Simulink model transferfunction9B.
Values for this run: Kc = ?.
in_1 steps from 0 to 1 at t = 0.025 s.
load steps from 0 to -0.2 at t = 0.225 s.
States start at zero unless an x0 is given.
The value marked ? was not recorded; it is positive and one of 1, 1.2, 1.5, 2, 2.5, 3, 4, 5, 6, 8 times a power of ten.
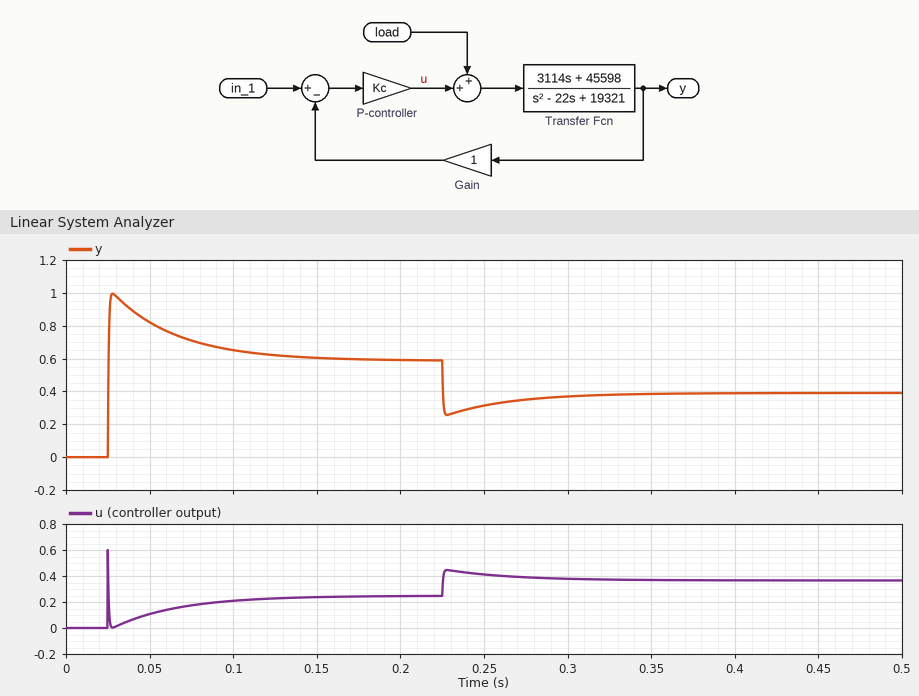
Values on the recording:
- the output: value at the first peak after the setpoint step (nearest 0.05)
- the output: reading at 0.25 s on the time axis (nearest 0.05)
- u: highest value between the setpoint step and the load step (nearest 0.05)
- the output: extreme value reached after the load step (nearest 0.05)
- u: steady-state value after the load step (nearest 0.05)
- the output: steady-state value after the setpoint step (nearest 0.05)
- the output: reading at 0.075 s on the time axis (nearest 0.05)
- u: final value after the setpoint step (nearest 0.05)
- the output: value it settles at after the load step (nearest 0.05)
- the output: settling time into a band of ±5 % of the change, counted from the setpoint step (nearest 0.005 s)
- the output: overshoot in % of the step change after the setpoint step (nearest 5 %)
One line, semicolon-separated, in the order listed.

1.00; 0.30; 0.60; 0.25; 0.35; 0.60; 0.70; 0.25; 0.40; 0.105 s; 70 %
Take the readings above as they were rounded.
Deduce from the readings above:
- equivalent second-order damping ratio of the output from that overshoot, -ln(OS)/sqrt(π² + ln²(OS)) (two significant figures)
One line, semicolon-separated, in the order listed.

0.11
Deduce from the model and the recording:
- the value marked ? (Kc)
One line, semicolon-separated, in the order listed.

0.6
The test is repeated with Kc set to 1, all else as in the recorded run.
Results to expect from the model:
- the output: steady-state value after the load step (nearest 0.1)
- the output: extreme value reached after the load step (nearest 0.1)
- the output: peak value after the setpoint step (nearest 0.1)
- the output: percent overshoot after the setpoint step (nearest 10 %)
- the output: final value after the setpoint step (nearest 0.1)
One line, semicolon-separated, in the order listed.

0.6; 0.5; 1.0; 40 %; 0.7
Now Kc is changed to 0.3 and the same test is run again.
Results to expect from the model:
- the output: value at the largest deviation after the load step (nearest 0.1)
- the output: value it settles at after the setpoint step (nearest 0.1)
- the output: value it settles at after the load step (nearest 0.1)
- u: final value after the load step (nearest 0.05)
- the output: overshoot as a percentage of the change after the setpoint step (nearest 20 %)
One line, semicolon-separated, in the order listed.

-0.2; 0.4; 0.1; 0.25; 140 %
